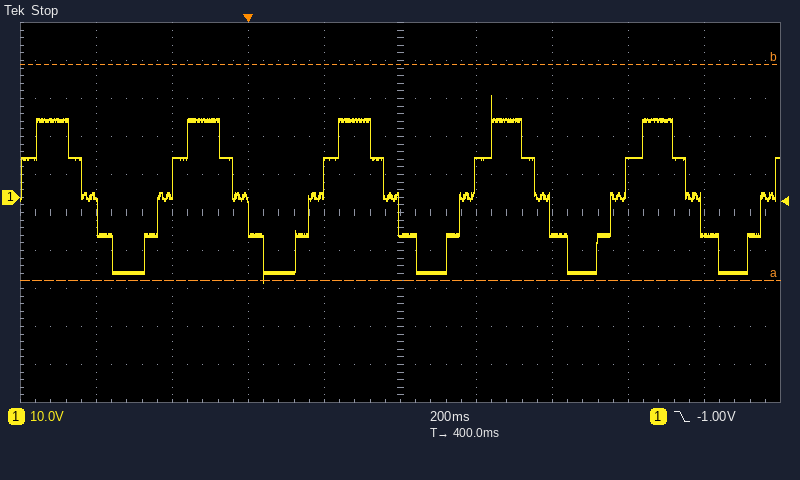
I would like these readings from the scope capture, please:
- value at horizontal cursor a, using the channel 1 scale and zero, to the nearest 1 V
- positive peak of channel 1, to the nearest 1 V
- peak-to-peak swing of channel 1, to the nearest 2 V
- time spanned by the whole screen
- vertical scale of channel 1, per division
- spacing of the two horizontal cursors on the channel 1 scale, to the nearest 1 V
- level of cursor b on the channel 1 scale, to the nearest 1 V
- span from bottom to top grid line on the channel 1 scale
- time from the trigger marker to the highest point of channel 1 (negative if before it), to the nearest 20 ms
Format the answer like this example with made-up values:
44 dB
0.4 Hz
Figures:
-22 V
27 V
50 V
2 s
10 V
57 V
35 V
100 V
+640 ms
